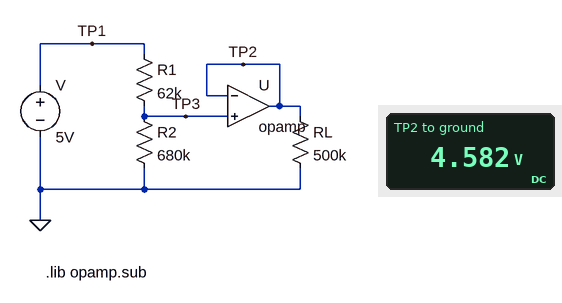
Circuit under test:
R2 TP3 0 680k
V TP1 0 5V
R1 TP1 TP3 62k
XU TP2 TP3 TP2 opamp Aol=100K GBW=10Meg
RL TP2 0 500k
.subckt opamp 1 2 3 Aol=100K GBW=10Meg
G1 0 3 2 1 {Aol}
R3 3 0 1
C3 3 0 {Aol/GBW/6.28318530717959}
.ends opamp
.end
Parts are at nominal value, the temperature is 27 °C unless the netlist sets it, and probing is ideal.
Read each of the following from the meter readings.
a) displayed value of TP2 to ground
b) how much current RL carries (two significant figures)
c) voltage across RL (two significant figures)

4.582 V
9.2 µA
4.6 V
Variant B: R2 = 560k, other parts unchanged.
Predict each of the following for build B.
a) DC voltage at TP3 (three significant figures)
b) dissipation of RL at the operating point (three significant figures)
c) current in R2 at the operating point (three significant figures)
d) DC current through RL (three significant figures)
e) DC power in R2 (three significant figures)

4.50 V
40.5 µW
8.04 µA
9.00 µA
36.2 µW
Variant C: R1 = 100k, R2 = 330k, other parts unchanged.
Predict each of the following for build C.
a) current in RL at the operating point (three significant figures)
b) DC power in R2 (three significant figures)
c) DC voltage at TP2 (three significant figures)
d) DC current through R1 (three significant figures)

7.67 µA
44.6 µW
3.84 V
11.6 µA
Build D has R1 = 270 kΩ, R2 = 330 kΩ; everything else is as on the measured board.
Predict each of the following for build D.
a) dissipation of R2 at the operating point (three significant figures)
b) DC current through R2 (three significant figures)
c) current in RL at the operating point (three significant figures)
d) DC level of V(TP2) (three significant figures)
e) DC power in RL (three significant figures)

22.9 µW
8.33 µA
5.50 µA
2.75 V
15.1 µW
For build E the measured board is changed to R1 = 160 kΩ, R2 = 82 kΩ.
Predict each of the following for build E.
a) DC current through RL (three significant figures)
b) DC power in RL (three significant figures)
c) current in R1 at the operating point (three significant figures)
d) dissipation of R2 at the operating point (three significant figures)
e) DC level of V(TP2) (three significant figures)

3.39 µA
5.74 µW
20.7 µA
35.0 µW
1.69 V
